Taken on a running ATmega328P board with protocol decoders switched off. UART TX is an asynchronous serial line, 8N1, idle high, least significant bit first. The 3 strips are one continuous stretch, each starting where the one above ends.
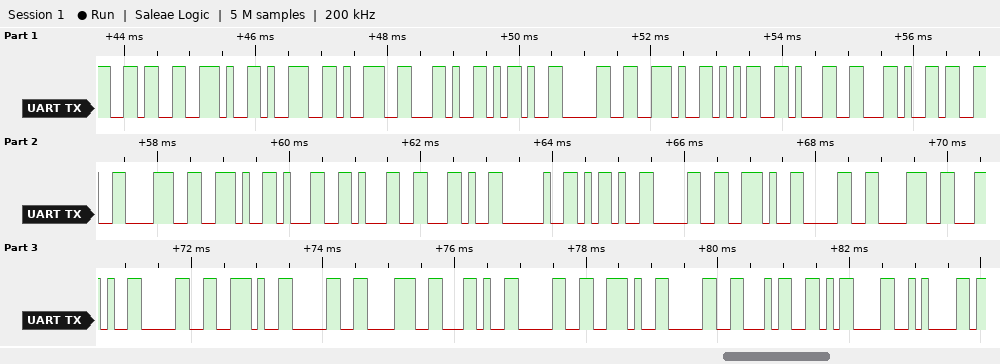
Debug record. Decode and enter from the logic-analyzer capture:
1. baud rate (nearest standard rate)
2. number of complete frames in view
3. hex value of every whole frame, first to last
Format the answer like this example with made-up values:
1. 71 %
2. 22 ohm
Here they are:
1. 9600 baud
2. 35
3. 36 2E 39 39 2C 2D 30 2E 35 31 2C 33 38 2E 31 31 2C 20 2D 30 2E 30 38 2C 30 2E 30 38 2C 30 2E 30 34 0D 0A
